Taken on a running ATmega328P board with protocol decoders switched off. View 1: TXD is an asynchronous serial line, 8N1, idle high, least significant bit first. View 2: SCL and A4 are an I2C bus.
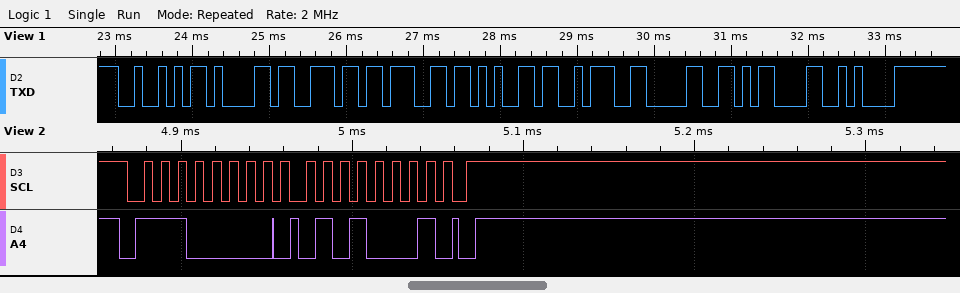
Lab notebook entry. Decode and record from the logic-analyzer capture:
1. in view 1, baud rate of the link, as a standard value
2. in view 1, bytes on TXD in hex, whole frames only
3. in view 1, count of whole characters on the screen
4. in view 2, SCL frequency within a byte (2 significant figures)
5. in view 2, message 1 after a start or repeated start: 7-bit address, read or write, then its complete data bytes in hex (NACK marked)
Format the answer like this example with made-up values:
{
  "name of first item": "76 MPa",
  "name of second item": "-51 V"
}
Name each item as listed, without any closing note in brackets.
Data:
{
  "in view 1, baud rate of the link, as a standard value": "9600 baud",
  "in view 1, bytes on TXD in hex, whole frames only": "0x52 0x61 0x6E 0x67 0x65 0x3A 0x30 0x0D 0x0A",
  "in view 1, count of whole characters on the screen": "9",
  "in view 2, SCL frequency within a byte": "100 kHz",
  "in view 2, message 1 after a start or repeated start: 7-bit address, read or write, then its complete data bytes in hex": "0x70 write: 51"
}
